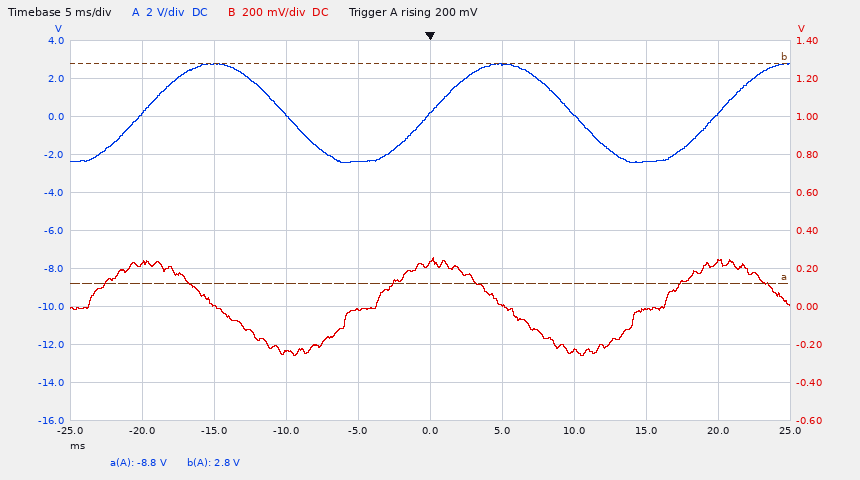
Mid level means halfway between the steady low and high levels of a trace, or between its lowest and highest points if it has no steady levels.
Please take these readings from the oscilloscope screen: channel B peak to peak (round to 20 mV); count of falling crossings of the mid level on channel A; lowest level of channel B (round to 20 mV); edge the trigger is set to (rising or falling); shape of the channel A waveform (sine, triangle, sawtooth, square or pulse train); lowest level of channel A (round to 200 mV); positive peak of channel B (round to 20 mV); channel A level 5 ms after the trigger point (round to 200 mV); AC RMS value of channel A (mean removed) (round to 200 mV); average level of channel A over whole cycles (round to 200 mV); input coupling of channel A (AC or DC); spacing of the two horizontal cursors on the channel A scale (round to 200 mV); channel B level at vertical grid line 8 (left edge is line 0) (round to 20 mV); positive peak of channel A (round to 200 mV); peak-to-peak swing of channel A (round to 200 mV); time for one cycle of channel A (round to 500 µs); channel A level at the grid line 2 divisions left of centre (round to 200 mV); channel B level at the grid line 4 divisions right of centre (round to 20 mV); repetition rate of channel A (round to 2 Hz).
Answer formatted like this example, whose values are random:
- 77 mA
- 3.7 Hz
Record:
- 520 mV
- 2
- -260 mV
- rising
- sine
- -2.4 V
- 260 mV
- 2.8 V
- 1.8 V
- 200 mV
- DC
- 11.6 V
- -20 mV
- 2.8 V
- 5.2 V
- 20.0 ms
- 0.0 V
- 240 mV
- 50 Hz
